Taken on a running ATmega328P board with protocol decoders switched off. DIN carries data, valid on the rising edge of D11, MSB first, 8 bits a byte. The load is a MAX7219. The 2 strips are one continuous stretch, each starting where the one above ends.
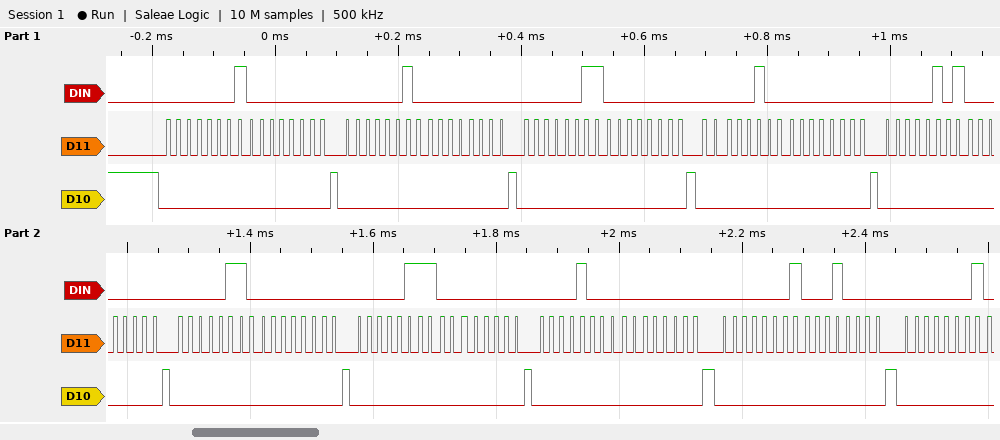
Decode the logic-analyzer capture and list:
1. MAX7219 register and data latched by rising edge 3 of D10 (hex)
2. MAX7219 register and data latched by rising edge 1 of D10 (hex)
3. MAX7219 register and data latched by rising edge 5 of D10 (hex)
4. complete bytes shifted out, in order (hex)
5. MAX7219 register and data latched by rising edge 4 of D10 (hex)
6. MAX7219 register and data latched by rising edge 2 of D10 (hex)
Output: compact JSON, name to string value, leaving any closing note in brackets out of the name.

{"MAX7219 register and data latched by rising edge 3 of D10": "register 0x3, data 0x00", "MAX7219 register and data latched by rising edge 1 of D10": "register 0x1, data 0x00", "MAX7219 register and data latched by rising edge 5 of D10": "register 0x5, data 0x00", "complete bytes shifted out, in order": "01 00 02 00 03 00 04 00 05 00 06 00 07 00 08 00 01 10 01", "MAX7219 register and data latched by rising edge 4 of D10": "register 0x4, data 0x00", "MAX7219 register and data latched by rising edge 2 of D10": "register 0x2, data 0x00"}
